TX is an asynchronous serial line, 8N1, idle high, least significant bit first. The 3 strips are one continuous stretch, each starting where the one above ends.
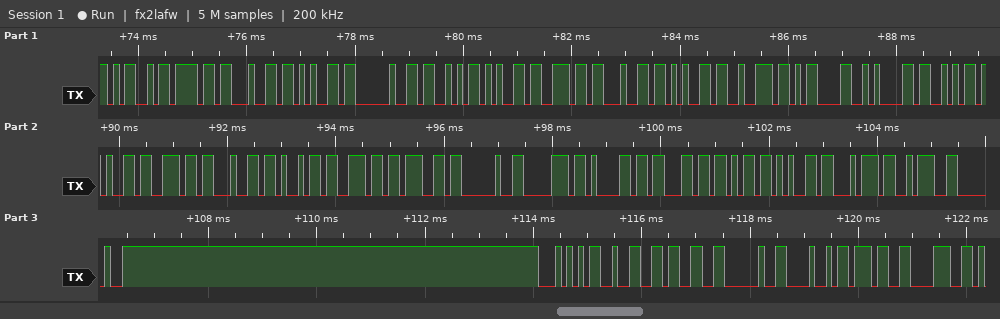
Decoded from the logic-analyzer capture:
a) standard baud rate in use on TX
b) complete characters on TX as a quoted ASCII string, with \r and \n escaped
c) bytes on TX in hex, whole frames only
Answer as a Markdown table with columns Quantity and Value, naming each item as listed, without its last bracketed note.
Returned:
| Quantity | Value |
|---|---|
| standard baud rate in use on TX | 9600 baud |
| complete characters on TX as a quoted ASCII string, with \r and \n escaped | "Mode Sender\r\nSending packet: T23 H78" |
| bytes on TX in hex, whole frames only | 4D 6F 64 65 20 53 65 6E 64 65 72 0D 0A 53 65 6E 64 69 6E 67 20 70 61 63 6B 65 74 3A 20 54 32 33 20 48 37 38 |
